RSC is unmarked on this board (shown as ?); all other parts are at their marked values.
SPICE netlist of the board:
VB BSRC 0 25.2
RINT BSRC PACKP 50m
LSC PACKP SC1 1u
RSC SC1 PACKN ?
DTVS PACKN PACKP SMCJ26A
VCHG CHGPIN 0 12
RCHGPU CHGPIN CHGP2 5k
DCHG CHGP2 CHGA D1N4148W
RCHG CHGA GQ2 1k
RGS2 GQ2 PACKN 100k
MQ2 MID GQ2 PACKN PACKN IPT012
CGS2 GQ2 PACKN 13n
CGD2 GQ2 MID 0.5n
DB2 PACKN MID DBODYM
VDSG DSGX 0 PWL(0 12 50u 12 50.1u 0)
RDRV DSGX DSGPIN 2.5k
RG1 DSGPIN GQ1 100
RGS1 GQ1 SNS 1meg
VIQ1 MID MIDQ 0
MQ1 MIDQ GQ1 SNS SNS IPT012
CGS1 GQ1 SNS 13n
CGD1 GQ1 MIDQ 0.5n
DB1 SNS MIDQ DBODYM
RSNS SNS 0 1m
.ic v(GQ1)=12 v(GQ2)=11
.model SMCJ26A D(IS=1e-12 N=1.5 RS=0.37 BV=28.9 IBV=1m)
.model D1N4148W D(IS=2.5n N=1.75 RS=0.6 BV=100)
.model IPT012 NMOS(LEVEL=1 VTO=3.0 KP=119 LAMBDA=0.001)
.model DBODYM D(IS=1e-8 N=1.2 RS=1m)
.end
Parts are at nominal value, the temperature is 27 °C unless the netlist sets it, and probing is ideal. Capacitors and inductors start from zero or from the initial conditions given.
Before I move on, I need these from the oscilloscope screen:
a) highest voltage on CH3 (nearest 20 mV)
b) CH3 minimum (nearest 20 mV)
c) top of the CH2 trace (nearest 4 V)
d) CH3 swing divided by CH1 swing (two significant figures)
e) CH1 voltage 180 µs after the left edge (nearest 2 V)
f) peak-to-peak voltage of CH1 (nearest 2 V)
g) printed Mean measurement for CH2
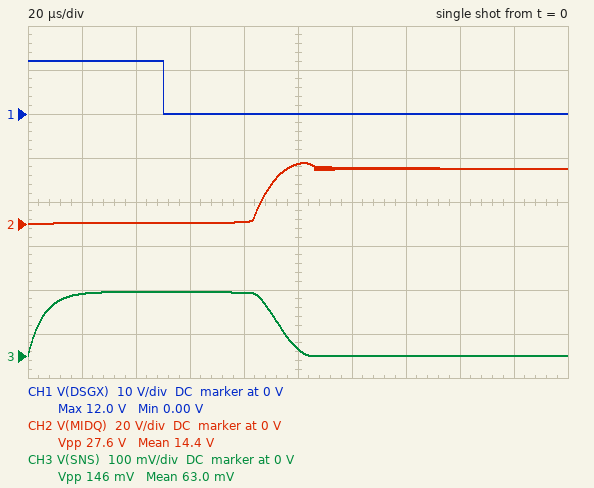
140 mV
0 V
28 V
0.012
0 V
12 V
14.4 V
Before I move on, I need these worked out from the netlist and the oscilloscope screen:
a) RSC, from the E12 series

0.12 Ω
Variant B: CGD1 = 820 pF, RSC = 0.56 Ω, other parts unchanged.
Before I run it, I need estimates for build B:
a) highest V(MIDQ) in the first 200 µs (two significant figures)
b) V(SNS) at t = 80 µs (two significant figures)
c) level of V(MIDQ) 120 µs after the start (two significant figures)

26 V
41 mV
25 V
